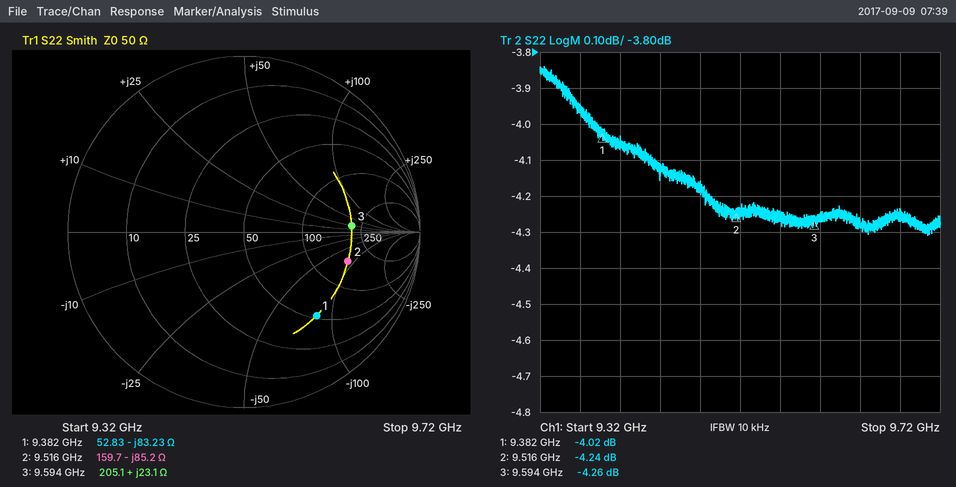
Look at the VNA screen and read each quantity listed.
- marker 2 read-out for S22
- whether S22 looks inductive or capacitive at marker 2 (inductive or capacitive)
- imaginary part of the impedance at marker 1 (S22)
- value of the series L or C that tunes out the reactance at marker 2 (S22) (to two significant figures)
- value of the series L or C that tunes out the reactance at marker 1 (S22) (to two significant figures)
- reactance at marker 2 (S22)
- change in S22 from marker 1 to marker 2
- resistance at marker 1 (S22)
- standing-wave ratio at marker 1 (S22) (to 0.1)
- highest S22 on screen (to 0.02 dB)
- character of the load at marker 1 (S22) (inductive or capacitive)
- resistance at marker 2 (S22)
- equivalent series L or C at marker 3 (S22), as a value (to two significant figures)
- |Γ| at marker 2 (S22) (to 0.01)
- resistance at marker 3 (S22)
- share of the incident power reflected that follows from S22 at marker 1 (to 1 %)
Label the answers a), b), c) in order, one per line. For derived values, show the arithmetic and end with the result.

a) -4.24 dB
b) capacitive
c) -83.23 Ω
d) L = 85.2 Ω/(2π × 9.516 GHz) ≈ 1.4 nH
e) L = 83.23 Ω/(2π × 9.382 GHz) ≈ 1.4 nH
f) -85.2 Ω
g) -4.24 − (-4.02) = -0.22 dB
h) 52.83 Ω
i) 4.4
j) -3.84 dB
k) capacitive
l) 159.7 Ω
m) L = 23.1 Ω/(2π × 9.594 GHz) ≈ 383 pH, so 380 pH to two significant figures
n) 0.61
o) 205.1 Ω
p) 10^(-4.02/10) ≈ 40 %
